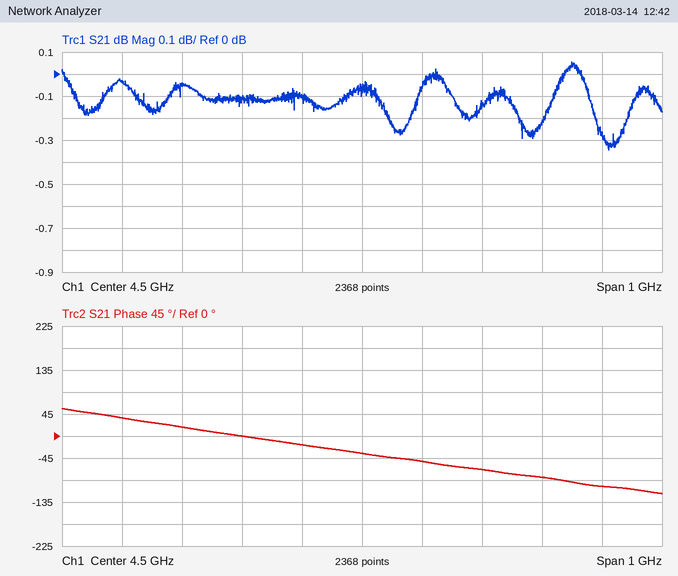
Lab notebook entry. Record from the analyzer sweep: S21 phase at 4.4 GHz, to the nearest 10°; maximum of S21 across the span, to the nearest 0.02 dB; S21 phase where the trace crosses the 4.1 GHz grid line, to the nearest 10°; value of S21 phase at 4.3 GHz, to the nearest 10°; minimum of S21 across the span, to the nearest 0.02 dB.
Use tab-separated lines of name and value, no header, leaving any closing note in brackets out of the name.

S21 phase at 4.4 GHz, to the nearest 10°	-20°
maximum of S21 across the span, to the nearest 0.02 dB	0.06 dB
S21 phase where the trace crosses the 4.1 GHz grid line, to the nearest 10°	40°
value of S21 phase at 4.3 GHz, to the nearest 10°	0°
minimum of S21 across the span, to the nearest 0.02 dB	-0.34 dB
